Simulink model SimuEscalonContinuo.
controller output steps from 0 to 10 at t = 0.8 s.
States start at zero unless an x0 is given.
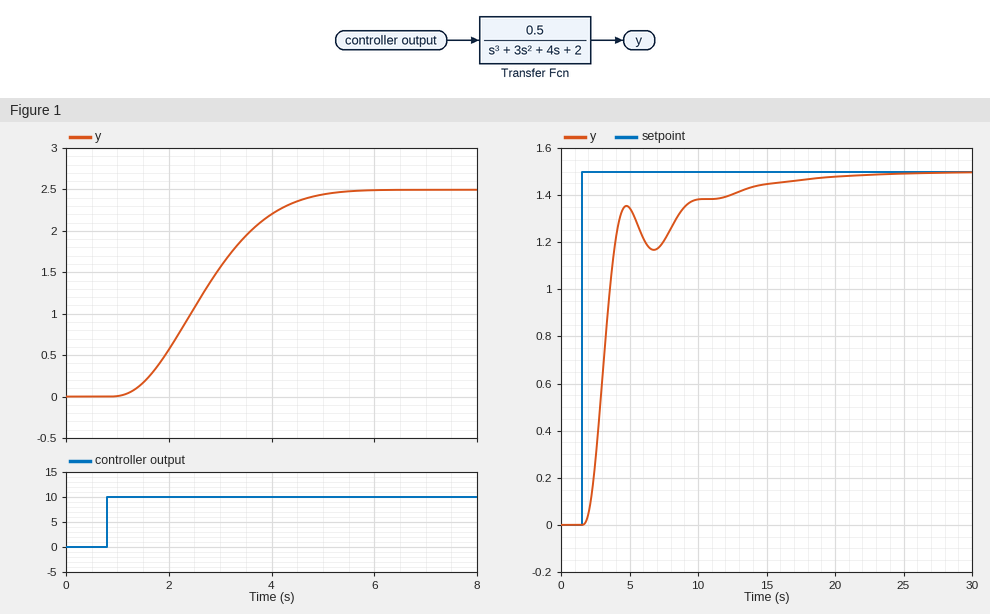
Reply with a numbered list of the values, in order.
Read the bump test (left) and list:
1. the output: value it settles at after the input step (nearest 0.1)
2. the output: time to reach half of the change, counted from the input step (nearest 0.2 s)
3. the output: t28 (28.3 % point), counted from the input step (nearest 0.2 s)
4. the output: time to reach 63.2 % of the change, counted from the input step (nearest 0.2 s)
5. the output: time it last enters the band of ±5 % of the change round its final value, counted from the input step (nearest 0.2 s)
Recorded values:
1. 2.5
2. 1.8 s
3. 1.4 s
4. 2.2 s
5. 3.8 s
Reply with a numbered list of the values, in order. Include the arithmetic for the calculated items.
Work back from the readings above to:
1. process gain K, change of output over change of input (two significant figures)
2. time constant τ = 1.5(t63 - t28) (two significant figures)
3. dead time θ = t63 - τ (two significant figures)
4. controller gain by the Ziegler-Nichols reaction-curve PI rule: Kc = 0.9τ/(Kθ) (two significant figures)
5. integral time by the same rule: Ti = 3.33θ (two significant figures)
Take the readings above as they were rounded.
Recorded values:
1. (2.5 - 0) / 10 = 0.25
2. 1.5 × (2.2 - 1.4) = 1.2 s
3. 2.2 - 1.2 = 1.0 s
4. 0.9 × 1.2 / (0.25 × 1) = 4.3
5. 3.33 × 1 = 3.3 s
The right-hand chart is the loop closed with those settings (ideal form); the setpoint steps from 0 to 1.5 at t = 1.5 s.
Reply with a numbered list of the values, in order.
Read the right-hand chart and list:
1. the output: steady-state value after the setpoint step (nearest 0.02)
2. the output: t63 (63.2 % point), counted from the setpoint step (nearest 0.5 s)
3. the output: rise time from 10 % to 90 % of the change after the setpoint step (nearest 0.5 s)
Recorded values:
1. 1.50
2. 2.0 s
3. 2.5 s
